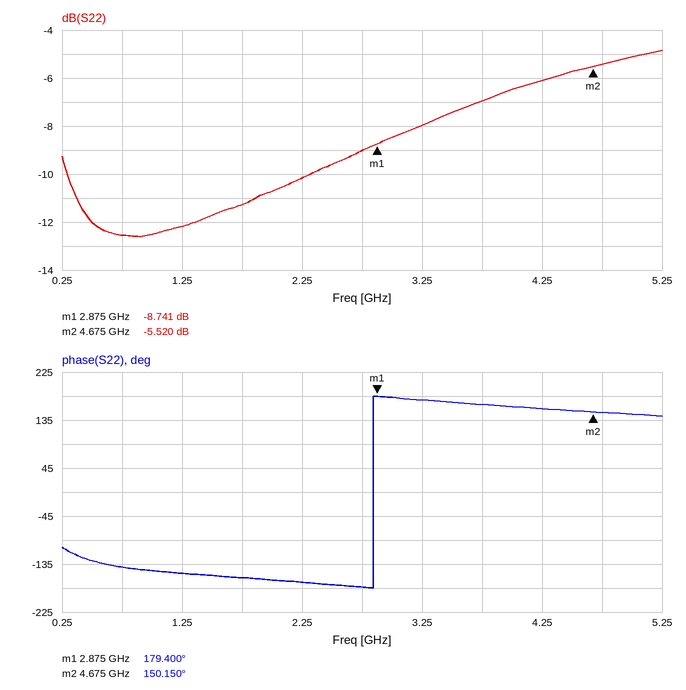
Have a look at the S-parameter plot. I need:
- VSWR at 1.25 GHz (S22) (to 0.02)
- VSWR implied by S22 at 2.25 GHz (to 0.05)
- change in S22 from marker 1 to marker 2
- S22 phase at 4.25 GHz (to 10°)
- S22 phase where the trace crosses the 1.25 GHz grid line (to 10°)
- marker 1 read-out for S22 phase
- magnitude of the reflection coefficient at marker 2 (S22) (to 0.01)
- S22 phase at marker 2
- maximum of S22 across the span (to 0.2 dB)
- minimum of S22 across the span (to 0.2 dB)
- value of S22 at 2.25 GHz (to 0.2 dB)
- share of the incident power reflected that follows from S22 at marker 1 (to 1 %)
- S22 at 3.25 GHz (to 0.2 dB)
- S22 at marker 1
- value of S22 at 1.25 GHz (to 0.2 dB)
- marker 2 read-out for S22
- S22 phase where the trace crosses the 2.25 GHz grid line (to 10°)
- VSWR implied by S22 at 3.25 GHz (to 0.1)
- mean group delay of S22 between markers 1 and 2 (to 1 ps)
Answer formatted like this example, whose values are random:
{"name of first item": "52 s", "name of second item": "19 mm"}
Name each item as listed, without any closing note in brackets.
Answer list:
{"VSWR at 1.25 GHz (S22)": "1.66", "VSWR implied by S22 at 2.25 GHz": "1.90", "change in S22 from marker 1 to marker 2": "3.221 dB", "S22 phase at 4.25 GHz": "160°", "S22 phase where the trace crosses the 1.25 GHz grid line": "-150°", "marker 1 read-out for S22 phase": "179.400°", "magnitude of the reflection coefficient at marker 2 (S22)": "0.53", "S22 phase at marker 2": "150.150°", "maximum of S22 across the span": "-4.8 dB", "minimum of S22 across the span": "-12.6 dB", "value of S22 at 2.25 GHz": "-10.2 dB", "share of the incident power reflected that follows from S22 at marker 1": "13 %", "S22 at 3.25 GHz": "-8.0 dB", "S22 at marker 1": "-8.741 dB", "value of S22 at 1.25 GHz": "-12.2 dB", "marker 2 read-out for S22": "-5.520 dB", "S22 phase where the trace crosses the 2.25 GHz grid line": "-170°", "VSWR implied by S22 at 3.25 GHz": "2.3", "mean group delay of S22 between markers 1 and 2": "45 ps"}
